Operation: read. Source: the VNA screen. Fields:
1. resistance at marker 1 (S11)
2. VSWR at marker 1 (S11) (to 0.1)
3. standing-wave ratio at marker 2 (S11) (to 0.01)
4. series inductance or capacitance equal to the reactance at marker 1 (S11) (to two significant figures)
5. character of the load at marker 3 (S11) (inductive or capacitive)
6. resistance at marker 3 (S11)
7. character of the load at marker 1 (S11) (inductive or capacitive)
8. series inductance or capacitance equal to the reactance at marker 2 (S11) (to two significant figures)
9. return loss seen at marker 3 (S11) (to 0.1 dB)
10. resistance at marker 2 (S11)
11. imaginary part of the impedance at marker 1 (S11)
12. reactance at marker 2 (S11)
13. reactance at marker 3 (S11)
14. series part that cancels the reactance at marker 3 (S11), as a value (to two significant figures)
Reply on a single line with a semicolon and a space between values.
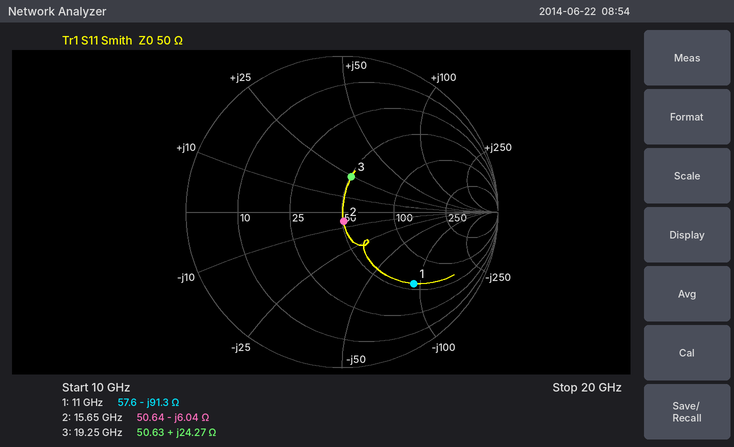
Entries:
57.6 Ω; 4.7; 1.13; 160 fF; inductive; 50.63 Ω; capacitive; 1.7 pF; 12.6 dB; 50.64 Ω; -91.3 Ω; -6.04 Ω; +24.27 Ω; 340 fF
